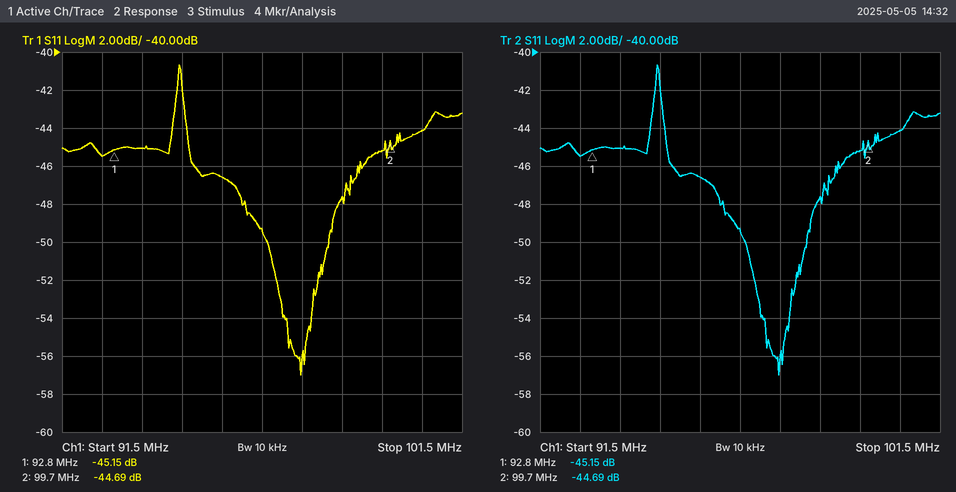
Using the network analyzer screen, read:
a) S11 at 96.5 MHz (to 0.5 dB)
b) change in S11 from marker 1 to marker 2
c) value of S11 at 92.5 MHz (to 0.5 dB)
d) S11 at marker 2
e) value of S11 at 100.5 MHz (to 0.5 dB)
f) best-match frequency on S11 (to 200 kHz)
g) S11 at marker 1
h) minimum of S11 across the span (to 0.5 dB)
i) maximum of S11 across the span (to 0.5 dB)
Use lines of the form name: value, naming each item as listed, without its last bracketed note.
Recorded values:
S11 at 96.5 MHz: -49.5 dB
change in S11 from marker 1 to marker 2: 0.46 dB
value of S11 at 92.5 MHz: -45.5 dB
S11 at marker 2: -44.69 dB
value of S11 at 100.5 MHz: -44.0 dB
best-match frequency on S11: 97.4 MHz
S11 at marker 1: -45.15 dB
minimum of S11 across the span: -57.0 dB
maximum of S11 across the span: -40.5 dB
